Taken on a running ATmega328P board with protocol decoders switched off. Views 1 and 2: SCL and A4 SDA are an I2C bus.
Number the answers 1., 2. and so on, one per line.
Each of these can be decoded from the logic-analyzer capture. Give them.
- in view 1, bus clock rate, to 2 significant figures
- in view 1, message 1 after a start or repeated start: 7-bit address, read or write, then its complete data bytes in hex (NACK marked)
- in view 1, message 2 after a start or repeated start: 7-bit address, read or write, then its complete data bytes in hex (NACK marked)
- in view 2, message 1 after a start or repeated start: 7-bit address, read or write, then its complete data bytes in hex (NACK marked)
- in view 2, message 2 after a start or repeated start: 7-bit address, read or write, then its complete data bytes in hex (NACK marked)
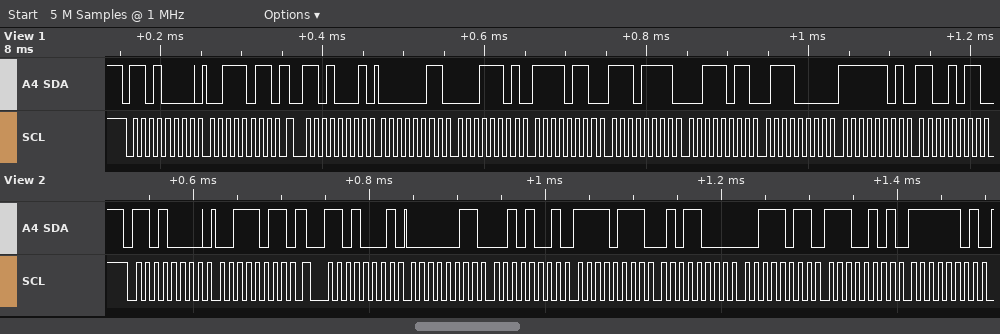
1. 100 kHz
2. 0x68 write: 3B
3. 0x68 read: 03 1D F6 EF 3B 70 FD CB
4. 0x68 write: 3B
5. 0x68 read: 03 29 F7 58 3B E5 FD
